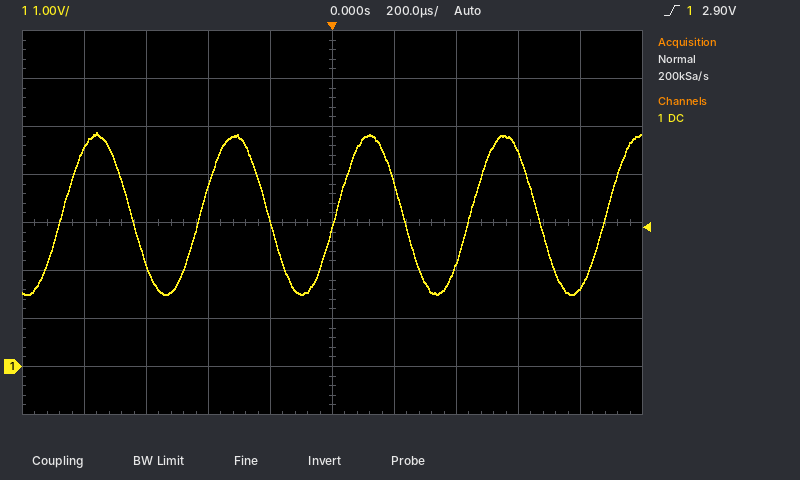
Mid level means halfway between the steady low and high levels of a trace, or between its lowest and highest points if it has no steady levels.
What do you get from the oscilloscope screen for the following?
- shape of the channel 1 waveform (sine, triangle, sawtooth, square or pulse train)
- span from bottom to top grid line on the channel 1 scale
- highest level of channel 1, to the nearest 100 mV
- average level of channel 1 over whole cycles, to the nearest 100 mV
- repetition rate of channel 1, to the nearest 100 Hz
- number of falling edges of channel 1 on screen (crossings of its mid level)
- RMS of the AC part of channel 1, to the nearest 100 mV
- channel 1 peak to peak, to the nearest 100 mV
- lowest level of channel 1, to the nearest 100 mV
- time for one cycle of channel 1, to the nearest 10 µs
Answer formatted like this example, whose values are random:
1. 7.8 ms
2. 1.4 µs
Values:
1. sine
2. 8 V
3. 4.9 V
4. 3.2 V
5. 2.3 kHz
6. 4
7. 1.2 V
8. 3.4 V
9. 1.5 V
10. 440 µs
